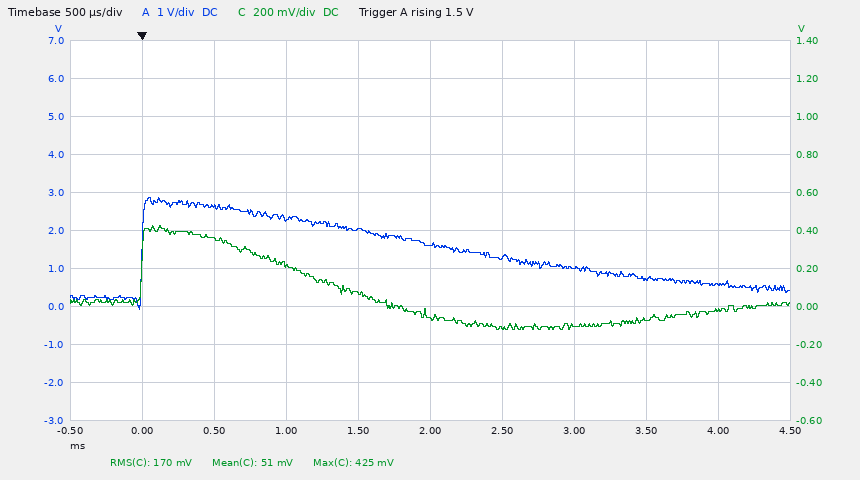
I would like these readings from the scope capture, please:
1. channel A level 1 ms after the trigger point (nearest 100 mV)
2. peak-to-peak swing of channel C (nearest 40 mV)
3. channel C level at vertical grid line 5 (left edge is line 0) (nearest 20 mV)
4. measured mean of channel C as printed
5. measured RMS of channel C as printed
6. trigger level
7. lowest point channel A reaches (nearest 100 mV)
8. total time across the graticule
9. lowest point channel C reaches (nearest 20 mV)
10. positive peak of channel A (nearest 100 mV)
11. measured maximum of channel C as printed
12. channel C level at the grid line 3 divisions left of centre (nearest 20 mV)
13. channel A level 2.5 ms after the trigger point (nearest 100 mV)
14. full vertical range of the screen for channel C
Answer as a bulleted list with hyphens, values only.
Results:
- 2.3 V
- 560 mV
- -60 mV
- 51 mV
- 170 mV
- 1.5 V
- -100 mV
- 5 ms
- -120 mV
- 2.9 V
- 425 mV
- 360 mV
- 1.3 V
- 2 V
